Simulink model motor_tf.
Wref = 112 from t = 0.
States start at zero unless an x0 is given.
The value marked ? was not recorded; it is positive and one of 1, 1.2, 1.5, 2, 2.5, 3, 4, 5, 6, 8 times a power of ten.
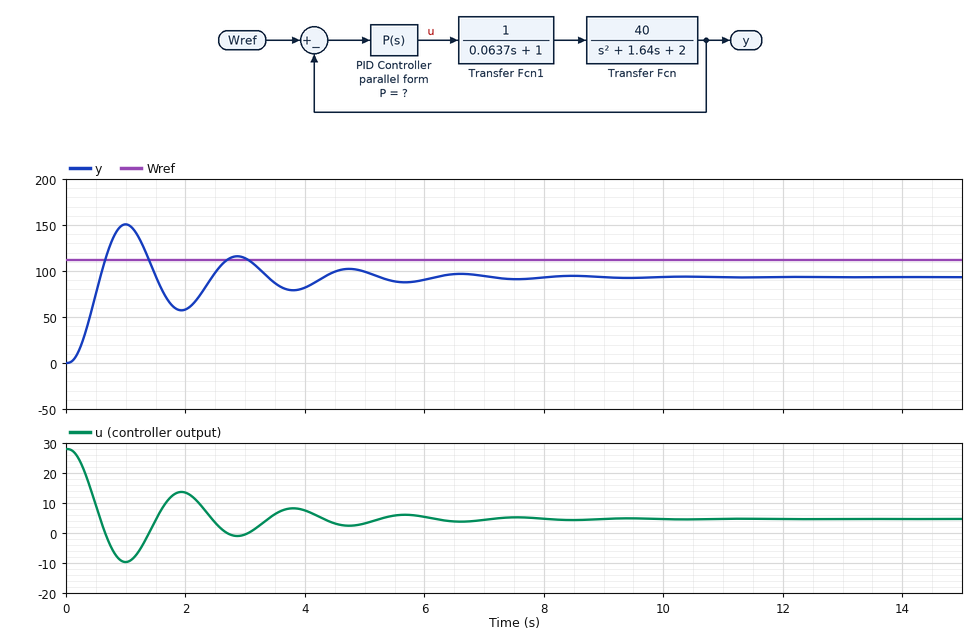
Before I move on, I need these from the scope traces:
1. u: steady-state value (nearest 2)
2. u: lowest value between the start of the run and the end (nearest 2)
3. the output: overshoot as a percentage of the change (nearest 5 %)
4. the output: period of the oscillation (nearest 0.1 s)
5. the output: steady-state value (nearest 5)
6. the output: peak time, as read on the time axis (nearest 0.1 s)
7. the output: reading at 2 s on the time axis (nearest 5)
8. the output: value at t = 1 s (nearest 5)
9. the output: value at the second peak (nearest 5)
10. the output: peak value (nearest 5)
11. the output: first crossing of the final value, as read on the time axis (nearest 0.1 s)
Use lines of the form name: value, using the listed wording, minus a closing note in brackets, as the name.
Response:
u: steady-state value: 4
u: lowest value between the start of the run and the end: -10
the output: overshoot as a percentage of the change: 60 %
the output: period of the oscillation: 1.9 s
the output: steady-state value: 95
the output: peak time, as read on the time axis: 1.0 s
the output: reading at 2 s on the time axis: 60
the output: value at t = 1 s: 150
the output: value at the second peak: 115
the output: peak value: 150
the output: first crossing of the final value, as read on the time axis: 0.6 s
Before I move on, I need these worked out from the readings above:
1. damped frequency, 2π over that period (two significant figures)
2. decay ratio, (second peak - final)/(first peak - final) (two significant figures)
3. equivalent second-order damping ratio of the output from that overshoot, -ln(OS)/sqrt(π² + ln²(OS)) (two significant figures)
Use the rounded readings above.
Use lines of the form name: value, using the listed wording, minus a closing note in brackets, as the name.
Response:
damped frequency, 2π over that period: 3.3 rad/s
decay ratio, (second peak - final)/(first peak - final): 0.36
equivalent second-order damping ratio of the output from that overshoot, -ln(OS)/sqrt(π² + ln²(OS)): 0.16
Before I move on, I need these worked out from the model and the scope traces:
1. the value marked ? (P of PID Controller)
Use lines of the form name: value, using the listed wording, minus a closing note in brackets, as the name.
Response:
the value marked ?: 0.25
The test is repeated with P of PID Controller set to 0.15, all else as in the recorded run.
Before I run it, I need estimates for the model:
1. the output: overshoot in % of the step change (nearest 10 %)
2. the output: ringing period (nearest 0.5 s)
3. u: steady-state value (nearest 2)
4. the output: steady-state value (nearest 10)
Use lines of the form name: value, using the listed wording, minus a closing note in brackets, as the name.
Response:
the output: overshoot in % of the step change: 50 %
the output: ringing period: 2.5 s
u: steady-state value: 4
the output: steady-state value: 80
